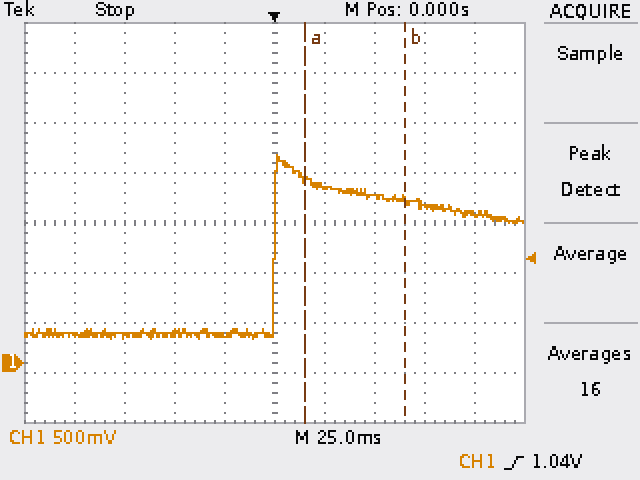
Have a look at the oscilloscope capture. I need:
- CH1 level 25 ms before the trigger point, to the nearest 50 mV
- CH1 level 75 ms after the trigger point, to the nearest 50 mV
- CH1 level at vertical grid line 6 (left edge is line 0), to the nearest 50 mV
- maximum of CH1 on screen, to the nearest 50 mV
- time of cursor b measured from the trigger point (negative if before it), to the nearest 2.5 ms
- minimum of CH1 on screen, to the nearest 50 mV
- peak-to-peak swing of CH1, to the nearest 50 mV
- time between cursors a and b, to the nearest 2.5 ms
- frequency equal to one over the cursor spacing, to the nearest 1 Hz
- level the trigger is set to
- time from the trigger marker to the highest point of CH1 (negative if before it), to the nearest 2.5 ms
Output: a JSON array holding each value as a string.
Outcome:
["300 mV", "1.60 V", "1.75 V", "2.10 V", "+65.0 ms", "250 mV", "1.85 V", "50.0 ms", "20 Hz", "1.04 V", "+2.5 ms"]
